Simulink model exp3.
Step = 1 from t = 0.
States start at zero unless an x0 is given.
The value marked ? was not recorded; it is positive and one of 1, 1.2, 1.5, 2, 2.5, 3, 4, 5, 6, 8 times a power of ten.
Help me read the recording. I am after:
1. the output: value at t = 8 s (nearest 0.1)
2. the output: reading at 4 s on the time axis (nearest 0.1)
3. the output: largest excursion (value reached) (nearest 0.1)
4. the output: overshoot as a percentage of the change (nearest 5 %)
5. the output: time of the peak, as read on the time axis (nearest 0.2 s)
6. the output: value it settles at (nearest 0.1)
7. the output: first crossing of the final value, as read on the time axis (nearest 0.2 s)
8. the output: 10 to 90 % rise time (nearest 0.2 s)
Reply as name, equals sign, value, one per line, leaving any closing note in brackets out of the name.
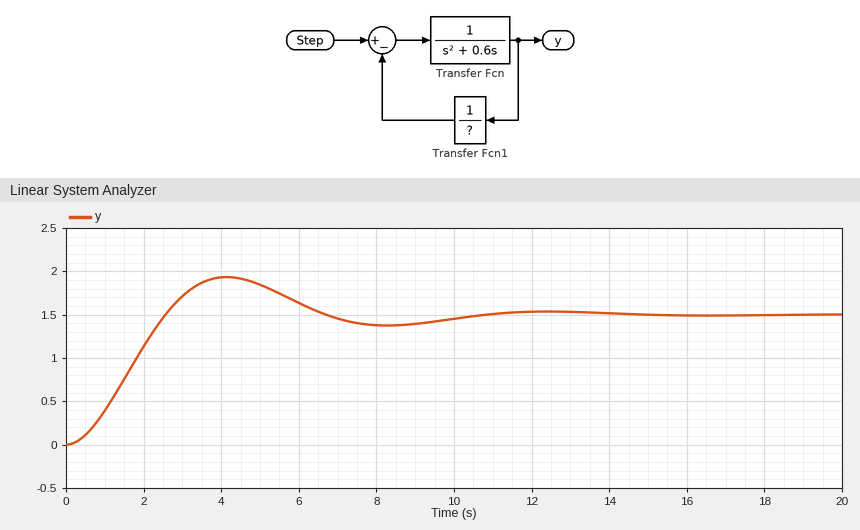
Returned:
the output: value at t = 8 s = 1.4
the output: reading at 4 s on the time axis = 1.9
the output: largest excursion (value reached) = 1.9
the output: overshoot as a percentage of the change = 30 %
the output: time of the peak, as read on the time axis = 4.2 s
the output: value it settles at = 1.5
the output: first crossing of the final value, as read on the time axis = 2.6 s
the output: 10 to 90 % rise time = 1.8 s
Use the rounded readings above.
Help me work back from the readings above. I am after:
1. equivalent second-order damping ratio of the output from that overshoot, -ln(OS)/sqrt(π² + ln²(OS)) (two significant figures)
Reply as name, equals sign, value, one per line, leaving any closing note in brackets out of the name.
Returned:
equivalent second-order damping ratio of the output from that overshoot, -ln(OS)/sqrt(π² + ln²(OS)) = 0.36
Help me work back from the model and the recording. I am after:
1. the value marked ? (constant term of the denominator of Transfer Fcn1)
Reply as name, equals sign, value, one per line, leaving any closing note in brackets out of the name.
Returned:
the value marked ? = 1.5
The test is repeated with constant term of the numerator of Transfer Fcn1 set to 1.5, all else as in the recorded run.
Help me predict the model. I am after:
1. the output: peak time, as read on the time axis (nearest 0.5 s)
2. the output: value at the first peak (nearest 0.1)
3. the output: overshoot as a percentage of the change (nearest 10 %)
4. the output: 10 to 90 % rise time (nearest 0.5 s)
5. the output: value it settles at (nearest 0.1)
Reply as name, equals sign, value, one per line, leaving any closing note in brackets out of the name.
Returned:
the output: peak time, as read on the time axis = 3.5 s
the output: value at the first peak = 1.4
the output: overshoot as a percentage of the change = 40 %
the output: 10 to 90 % rise time = 1.5 s
the output: value it settles at = 1.0
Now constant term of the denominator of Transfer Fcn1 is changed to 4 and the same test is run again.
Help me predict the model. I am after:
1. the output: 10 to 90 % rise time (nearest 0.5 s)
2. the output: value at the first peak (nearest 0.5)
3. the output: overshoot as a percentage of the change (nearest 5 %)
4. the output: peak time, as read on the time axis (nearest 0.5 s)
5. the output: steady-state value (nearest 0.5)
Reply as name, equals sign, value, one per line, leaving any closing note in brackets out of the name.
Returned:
the output: 10 to 90 % rise time = 3.5 s
the output: value at the first peak = 4.5
the output: overshoot as a percentage of the change = 10 %
the output: peak time, as read on the time axis = 8.0 s
the output: steady-state value = 4.0
